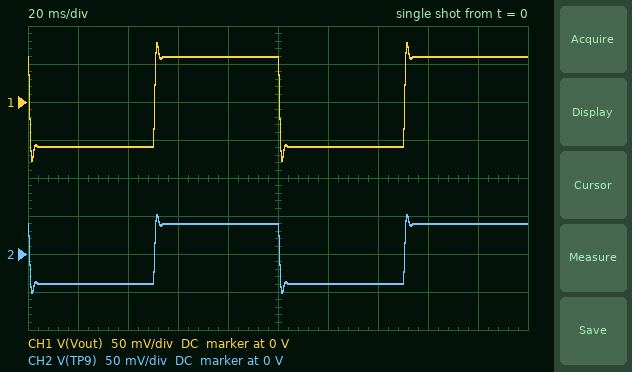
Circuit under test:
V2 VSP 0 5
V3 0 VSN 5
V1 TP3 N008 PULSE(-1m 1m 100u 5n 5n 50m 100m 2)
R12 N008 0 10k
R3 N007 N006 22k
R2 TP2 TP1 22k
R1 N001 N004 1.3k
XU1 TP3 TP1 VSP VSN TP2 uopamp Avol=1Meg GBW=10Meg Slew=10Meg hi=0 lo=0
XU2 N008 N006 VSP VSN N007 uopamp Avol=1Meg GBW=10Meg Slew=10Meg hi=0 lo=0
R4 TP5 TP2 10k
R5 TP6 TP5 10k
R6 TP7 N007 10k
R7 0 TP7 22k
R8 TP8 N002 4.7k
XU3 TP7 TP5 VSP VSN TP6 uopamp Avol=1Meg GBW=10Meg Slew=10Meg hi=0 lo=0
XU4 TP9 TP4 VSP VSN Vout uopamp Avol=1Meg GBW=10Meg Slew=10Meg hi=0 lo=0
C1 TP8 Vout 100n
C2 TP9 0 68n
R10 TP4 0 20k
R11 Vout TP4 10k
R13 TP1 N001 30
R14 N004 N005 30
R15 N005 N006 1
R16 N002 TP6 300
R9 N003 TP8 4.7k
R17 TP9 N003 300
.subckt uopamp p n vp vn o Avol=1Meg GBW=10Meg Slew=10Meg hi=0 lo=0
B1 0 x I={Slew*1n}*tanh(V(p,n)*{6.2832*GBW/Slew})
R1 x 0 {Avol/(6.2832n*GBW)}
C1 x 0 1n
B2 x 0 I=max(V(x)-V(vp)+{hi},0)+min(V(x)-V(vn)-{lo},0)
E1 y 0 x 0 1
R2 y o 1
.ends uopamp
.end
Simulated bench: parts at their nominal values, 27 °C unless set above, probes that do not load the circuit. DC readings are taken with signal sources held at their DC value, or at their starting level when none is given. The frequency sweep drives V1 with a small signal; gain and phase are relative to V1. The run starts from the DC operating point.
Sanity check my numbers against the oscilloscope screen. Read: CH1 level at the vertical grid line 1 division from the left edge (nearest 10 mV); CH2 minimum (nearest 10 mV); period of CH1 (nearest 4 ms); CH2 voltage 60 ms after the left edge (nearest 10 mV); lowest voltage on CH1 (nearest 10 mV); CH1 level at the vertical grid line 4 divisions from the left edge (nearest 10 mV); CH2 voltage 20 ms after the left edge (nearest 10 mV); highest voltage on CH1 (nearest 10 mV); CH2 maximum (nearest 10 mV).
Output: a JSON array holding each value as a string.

["-60 mV", "-50 mV", "100 ms", "40 mV", "-80 mV", "60 mV", "-40 mV", "80 mV", "50 mV"]
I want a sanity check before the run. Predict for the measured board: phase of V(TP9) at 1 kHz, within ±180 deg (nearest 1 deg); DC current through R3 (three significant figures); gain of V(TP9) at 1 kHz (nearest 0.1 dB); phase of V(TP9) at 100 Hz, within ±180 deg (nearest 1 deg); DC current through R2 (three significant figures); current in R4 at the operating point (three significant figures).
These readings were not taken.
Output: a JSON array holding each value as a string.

["25 deg", "735 nA", "15.9 dB", "164 deg", "735 nA", "2.83 µA"]
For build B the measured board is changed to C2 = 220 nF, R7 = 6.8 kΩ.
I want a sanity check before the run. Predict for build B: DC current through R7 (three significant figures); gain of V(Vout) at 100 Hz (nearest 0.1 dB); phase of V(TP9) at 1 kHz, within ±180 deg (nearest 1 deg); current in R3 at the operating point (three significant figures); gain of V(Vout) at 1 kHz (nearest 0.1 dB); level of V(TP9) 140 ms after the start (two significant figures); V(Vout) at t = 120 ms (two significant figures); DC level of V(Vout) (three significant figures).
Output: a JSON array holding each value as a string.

["962 nA", "29.9 dB", "30 deg", "735 nA", "5.5 dB", "-30 mV", "-45 mV", "45.4 mV"]
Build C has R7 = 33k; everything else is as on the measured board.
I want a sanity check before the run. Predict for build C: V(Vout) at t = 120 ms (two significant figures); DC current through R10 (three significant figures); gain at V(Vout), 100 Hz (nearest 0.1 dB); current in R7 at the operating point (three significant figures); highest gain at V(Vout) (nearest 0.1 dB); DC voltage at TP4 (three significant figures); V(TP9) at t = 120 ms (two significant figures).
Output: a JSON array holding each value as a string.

["-63 mV", "2.10 µA", "36.2 dB", "376 nA", "37.0 dB", "42.0 mV", "-42 mV"]
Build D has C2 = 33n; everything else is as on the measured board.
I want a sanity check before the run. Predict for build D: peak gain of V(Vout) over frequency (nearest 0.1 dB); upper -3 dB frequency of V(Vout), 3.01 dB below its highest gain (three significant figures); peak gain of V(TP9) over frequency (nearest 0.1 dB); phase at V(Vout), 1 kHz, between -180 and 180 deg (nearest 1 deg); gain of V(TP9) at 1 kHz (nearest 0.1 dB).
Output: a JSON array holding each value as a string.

["46.6 dB", "616 Hz", "43.1 dB", "12 deg", "24.6 dB"]
